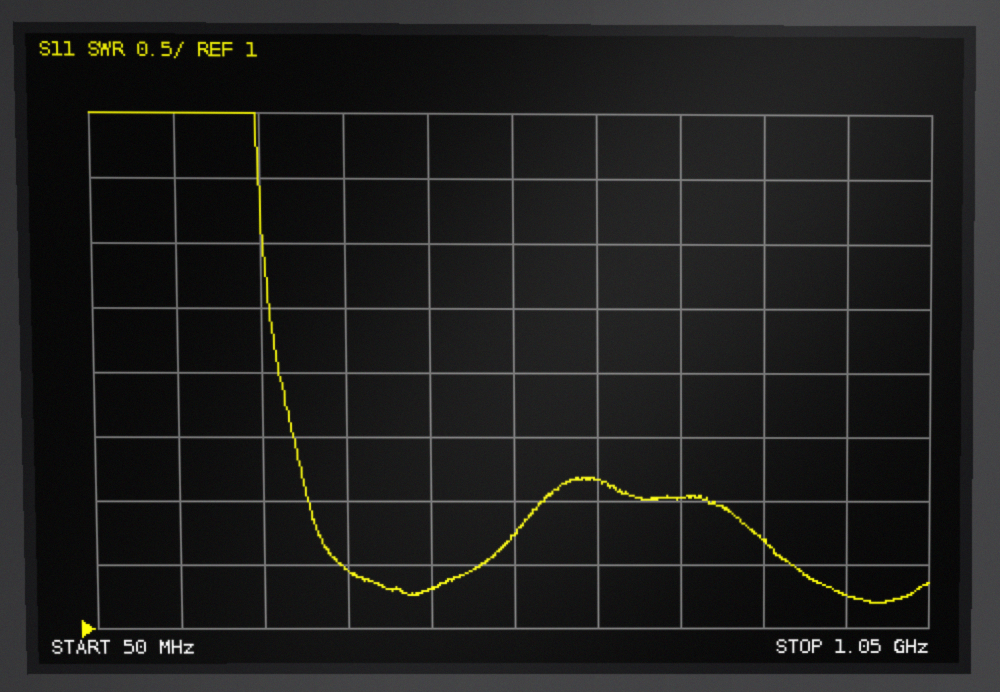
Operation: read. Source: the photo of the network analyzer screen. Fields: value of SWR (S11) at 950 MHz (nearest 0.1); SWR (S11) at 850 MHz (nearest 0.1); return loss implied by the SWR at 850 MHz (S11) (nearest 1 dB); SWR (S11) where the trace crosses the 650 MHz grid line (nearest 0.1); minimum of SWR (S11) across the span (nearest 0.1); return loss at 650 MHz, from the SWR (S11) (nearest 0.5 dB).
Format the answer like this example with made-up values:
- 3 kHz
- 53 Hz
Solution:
- 1.3
- 1.7
- 12 dB
- 2.2
- 1.2
- 8.5 dB
